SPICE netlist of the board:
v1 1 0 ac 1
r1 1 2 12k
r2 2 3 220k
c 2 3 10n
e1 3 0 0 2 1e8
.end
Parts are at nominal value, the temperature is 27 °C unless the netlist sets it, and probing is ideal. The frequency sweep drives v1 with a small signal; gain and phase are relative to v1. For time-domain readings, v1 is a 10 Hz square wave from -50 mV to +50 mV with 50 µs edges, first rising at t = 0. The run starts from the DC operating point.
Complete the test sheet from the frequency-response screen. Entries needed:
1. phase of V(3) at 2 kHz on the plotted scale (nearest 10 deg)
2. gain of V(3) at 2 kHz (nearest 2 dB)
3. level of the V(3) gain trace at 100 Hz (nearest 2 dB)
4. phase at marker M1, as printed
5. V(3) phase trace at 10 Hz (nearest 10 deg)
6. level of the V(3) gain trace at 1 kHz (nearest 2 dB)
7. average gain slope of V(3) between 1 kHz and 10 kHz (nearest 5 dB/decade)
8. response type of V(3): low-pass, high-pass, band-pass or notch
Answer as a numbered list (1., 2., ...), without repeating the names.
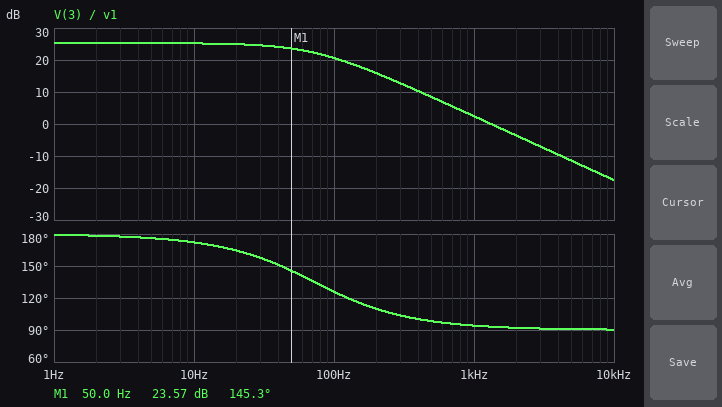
1. 90 deg
2. -4 dB
3. 20 dB
4. 145.3 deg
5. 170 deg
6. 2 dB
7. -20 dB/decade
8. low-pass
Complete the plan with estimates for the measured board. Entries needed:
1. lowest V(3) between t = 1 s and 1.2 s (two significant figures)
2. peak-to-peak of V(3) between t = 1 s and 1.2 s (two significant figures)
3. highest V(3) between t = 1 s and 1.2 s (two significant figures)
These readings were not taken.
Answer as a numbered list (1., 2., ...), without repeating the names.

1. -920 mV
2. 1.8 V
3. 920 mV
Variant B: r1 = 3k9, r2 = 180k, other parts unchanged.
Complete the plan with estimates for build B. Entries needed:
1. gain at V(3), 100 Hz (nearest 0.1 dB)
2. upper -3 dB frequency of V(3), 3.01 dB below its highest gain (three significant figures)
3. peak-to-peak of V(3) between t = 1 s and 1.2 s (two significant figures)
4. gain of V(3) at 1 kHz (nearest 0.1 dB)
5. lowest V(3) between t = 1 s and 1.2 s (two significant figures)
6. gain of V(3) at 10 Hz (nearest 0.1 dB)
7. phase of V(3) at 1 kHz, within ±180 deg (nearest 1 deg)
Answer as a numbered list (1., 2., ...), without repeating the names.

1. 29.7 dB
2. 88.4 Hz
3. 4.6 V
4. 12.2 dB
5. -2.3 V
6. 33.2 dB
7. 95 deg
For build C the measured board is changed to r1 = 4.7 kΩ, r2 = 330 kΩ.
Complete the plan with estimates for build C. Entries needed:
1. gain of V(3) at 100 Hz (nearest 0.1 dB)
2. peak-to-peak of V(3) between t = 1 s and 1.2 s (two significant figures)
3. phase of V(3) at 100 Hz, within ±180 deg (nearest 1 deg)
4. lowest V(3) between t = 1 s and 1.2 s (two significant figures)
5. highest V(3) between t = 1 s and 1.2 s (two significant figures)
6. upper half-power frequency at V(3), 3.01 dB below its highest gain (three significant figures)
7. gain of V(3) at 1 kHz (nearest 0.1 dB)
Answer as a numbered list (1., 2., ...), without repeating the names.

1. 29.7 dB
2. 7.0 V
3. 116 deg
4. -3.5 V
5. 3.5 V
6. 48.2 Hz
7. 10.6 dB
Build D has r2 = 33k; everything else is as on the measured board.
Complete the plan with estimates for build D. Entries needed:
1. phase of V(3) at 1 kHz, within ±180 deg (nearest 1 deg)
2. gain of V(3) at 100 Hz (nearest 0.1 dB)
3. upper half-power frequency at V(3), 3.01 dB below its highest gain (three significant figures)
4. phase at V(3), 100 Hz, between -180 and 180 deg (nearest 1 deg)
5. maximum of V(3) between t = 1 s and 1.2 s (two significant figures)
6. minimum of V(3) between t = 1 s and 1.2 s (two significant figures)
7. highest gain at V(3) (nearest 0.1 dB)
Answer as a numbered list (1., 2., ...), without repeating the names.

1. 116 deg
2. 8.6 dB
3. 482 Hz
4. 168 deg
5. 140 mV
6. -140 mV
7. 8.8 dB
